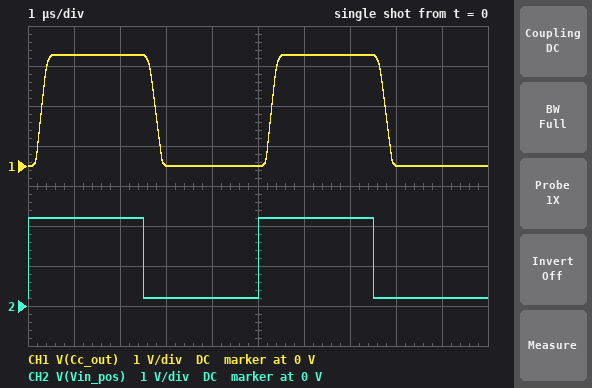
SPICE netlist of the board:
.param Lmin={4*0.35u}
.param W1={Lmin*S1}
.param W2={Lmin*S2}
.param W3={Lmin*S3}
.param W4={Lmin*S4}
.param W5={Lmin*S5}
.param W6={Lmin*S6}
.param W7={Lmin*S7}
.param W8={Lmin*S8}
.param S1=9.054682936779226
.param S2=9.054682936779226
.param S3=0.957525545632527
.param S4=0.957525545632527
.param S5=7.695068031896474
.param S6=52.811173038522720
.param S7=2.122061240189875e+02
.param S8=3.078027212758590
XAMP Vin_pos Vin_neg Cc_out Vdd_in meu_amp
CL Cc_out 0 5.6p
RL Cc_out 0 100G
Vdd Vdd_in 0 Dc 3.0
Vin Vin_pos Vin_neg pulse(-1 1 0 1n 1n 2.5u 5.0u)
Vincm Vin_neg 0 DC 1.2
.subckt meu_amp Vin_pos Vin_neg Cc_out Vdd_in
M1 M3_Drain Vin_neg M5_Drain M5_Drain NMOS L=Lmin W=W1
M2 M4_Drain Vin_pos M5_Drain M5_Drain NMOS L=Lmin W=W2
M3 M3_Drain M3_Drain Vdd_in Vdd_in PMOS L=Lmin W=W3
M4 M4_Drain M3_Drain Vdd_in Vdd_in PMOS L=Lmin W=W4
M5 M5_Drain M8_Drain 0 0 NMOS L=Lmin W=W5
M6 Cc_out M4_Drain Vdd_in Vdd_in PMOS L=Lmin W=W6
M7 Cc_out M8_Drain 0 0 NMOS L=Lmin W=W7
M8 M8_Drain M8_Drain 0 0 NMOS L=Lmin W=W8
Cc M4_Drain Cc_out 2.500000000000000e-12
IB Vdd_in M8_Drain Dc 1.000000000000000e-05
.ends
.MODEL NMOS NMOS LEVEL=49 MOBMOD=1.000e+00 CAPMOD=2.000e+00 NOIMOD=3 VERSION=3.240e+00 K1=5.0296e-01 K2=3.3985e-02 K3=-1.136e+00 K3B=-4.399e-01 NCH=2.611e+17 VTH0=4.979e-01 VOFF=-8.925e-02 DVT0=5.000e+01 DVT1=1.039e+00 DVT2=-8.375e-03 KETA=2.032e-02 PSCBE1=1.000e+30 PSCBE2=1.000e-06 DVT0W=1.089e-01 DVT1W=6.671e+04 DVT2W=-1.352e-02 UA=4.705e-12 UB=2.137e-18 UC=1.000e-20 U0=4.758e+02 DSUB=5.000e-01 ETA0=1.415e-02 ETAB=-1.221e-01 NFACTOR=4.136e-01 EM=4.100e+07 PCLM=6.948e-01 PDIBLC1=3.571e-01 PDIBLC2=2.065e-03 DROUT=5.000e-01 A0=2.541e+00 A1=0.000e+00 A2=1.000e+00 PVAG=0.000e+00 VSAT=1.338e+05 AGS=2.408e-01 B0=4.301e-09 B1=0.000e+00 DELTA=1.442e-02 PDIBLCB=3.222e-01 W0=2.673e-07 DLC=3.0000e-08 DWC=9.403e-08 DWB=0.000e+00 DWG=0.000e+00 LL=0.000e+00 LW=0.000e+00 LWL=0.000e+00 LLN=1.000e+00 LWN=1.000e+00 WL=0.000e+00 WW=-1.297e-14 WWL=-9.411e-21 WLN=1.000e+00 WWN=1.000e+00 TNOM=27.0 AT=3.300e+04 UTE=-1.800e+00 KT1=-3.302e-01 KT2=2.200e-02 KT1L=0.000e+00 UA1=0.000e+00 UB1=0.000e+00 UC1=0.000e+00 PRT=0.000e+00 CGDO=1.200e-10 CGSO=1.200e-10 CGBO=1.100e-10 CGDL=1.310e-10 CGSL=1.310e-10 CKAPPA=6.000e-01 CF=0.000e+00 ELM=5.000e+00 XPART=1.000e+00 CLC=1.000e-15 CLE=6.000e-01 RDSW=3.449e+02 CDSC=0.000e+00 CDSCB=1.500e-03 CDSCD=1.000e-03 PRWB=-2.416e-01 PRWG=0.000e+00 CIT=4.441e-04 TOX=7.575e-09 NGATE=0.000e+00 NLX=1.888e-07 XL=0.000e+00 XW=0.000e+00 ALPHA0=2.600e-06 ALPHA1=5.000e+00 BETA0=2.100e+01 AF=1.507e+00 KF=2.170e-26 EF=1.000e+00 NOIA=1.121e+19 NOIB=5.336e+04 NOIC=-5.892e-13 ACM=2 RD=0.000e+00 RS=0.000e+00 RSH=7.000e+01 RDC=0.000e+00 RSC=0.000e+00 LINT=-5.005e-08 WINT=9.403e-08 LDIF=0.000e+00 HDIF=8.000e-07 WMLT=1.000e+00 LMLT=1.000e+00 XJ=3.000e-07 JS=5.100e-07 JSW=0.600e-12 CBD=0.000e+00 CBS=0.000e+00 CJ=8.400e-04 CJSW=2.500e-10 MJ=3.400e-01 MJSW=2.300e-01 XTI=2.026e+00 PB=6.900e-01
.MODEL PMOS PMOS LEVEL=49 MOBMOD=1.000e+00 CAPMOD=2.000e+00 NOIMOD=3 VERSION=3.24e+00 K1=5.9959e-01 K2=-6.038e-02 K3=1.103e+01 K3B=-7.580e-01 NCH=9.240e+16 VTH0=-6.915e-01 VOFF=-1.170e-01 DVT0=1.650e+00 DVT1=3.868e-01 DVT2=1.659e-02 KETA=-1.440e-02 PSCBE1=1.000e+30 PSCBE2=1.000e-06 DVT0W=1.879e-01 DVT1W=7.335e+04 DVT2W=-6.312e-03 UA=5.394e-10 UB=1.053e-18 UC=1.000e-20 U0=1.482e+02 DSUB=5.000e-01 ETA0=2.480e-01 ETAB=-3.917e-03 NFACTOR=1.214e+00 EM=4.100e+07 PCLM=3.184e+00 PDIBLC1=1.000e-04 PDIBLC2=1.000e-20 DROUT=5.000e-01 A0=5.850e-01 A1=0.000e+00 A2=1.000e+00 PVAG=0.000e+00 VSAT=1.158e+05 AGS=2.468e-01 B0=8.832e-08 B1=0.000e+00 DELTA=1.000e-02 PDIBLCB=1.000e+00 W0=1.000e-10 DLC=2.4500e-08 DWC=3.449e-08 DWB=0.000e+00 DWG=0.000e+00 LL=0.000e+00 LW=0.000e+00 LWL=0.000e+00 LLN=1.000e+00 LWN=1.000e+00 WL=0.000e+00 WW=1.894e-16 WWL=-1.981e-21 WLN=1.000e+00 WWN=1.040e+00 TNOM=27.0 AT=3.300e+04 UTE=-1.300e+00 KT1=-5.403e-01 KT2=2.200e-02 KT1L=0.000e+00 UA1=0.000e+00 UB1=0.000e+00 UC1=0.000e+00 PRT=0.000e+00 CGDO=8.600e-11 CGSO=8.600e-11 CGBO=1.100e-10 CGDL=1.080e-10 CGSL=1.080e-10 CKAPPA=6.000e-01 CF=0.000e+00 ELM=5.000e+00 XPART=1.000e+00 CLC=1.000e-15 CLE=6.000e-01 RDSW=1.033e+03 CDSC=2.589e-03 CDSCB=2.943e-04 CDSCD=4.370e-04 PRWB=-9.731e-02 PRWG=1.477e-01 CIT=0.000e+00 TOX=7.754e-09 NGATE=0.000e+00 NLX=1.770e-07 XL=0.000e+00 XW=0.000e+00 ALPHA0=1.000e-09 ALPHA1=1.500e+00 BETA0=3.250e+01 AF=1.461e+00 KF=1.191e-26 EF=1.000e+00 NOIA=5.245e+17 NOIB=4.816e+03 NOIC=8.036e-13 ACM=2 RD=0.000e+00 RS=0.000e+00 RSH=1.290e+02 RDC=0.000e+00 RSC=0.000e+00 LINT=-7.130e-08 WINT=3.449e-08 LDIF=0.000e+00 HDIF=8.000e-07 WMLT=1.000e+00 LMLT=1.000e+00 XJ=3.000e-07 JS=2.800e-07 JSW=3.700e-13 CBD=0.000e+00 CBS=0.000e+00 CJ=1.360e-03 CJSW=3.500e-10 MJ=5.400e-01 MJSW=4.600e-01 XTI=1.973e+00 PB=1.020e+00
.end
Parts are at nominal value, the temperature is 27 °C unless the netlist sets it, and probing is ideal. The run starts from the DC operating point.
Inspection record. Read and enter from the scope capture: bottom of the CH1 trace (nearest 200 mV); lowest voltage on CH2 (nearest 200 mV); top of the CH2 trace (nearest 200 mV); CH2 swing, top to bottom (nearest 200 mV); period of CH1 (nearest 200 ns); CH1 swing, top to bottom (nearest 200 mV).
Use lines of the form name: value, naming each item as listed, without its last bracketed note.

bottom of the CH1 trace: 0 V
lowest voltage on CH2: 200 mV
top of the CH2 trace: 2.2 V
CH2 swing, top to bottom: 2.0 V
period of CH1: 5.0 µs
CH1 swing, top to bottom: 2.8 V
